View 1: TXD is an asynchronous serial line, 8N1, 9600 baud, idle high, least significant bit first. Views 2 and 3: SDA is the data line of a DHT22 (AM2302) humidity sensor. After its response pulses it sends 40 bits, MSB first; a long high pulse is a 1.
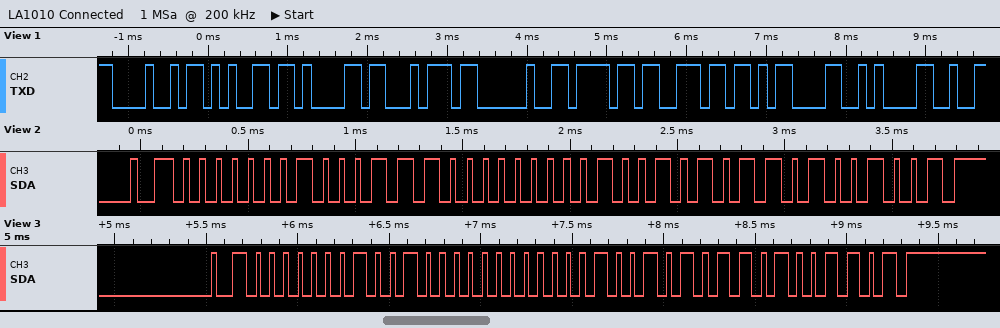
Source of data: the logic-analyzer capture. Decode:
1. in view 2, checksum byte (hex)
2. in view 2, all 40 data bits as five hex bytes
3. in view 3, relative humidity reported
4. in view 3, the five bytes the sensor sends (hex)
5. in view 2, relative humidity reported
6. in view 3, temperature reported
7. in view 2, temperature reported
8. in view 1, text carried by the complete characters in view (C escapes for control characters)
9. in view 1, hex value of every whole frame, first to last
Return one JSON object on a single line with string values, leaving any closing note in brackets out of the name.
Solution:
{"in view 2, checksum byte": "0x49", "in view 2, all 40 data bits as five hex bytes": "01 1C 01 2B 49", "in view 3, relative humidity reported": "28.8 %", "in view 3, the five bytes the sensor sends": "01 20 01 2B 4D", "in view 2, relative humidity reported": "28.4 %", "in view 3, temperature reported": "29.9 °C", "in view 2, temperature reported": "29.9 °C", "in view 1, text carried by the complete characters in view": "\"Heat on\\r\\n\"", "in view 1, hex value of every whole frame, first to last": "48 65 61 74 20 6F 6E 0D 0A"}
